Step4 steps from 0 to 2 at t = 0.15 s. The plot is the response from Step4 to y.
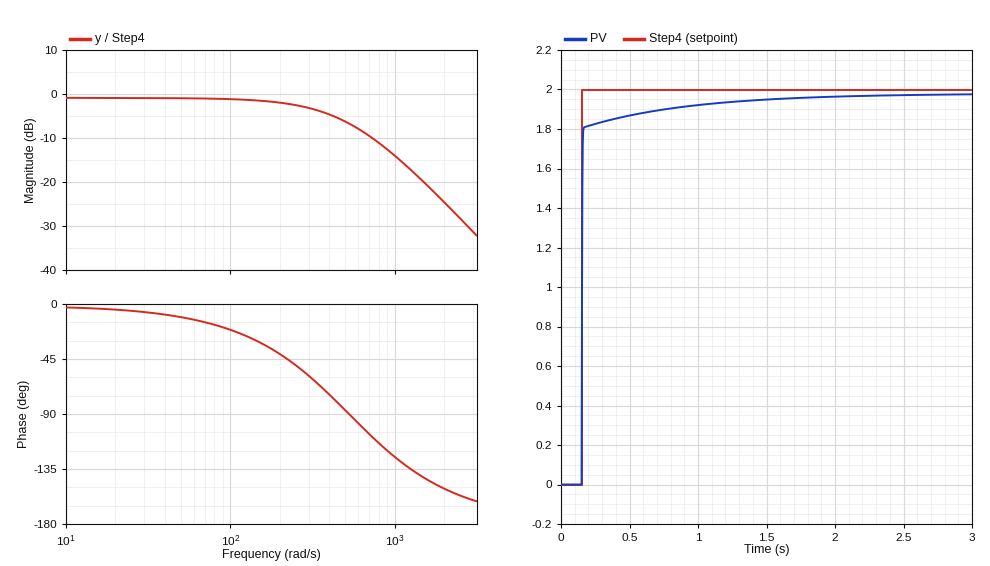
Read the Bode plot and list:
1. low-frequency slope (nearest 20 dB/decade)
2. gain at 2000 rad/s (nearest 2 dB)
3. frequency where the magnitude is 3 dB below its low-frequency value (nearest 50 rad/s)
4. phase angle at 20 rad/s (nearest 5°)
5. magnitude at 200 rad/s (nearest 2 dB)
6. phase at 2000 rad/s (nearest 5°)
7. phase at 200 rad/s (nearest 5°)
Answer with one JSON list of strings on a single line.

["0 dB/decade", "-24 dB", "350 rad/s", "-5°", "-2 dB", "-150°", "-40°"]
